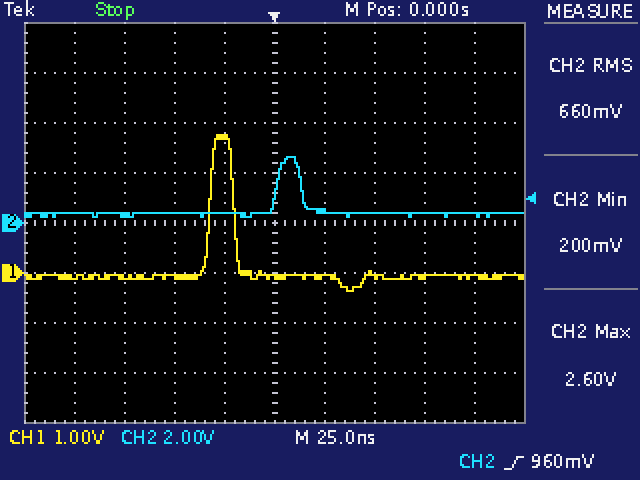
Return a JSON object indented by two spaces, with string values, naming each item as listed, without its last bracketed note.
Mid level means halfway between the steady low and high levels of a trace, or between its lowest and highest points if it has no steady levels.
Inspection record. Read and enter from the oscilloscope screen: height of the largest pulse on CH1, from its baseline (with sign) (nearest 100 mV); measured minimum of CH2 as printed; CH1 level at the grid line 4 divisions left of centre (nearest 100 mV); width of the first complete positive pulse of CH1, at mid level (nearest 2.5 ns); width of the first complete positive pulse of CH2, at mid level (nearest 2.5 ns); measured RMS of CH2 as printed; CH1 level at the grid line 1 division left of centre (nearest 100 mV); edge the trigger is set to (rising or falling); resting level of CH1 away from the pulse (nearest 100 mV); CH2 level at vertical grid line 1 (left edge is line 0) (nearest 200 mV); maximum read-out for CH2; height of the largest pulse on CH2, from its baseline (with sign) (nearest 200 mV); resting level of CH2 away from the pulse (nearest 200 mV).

{
  "height of the largest pulse on CH1, from its baseline (with sign)": "+2.8 V",
  "measured minimum of CH2 as printed": "200 mV",
  "CH1 level at the grid line 4 divisions left of centre": "-100 mV",
  "width of the first complete positive pulse of CH1, at mid level": "12.5 ns",
  "width of the first complete positive pulse of CH2, at mid level": "12.5 ns",
  "measured RMS of CH2 as printed": "660 mV",
  "CH1 level at the grid line 1 division left of centre": "2.7 V",
  "edge the trigger is set to": "rising",
  "resting level of CH1 away from the pulse": "-100 mV",
  "CH2 level at vertical grid line 1 (left edge is line 0)": "400 mV",
  "maximum read-out for CH2": "2.60 V",
  "height of the largest pulse on CH2, from its baseline (with sign)": "+2.2 V",
  "resting level of CH2 away from the pulse": "400 mV"
}
